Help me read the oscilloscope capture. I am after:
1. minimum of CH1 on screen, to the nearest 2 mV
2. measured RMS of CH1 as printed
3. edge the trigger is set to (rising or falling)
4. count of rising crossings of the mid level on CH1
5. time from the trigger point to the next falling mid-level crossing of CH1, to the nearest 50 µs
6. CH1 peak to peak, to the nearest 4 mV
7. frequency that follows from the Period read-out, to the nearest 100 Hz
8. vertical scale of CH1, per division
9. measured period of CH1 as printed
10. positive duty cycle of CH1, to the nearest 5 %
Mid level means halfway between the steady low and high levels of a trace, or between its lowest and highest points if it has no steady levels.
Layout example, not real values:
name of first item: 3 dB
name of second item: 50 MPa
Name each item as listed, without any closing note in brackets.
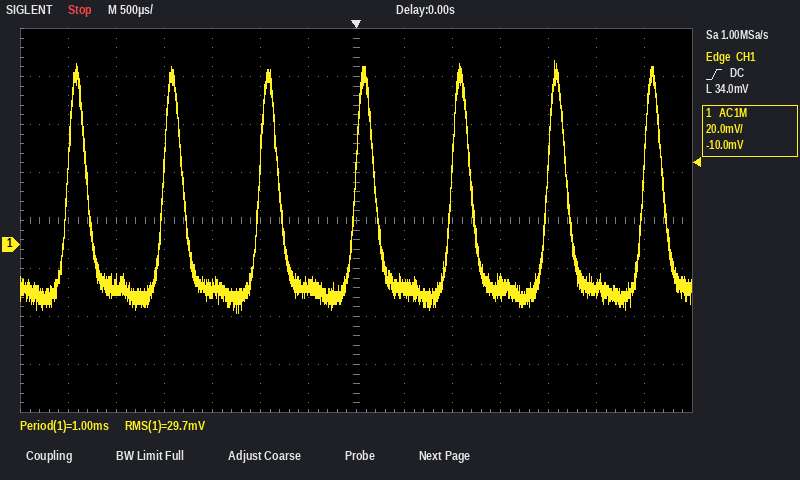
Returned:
minimum of CH1 on screen, to the nearest 2 mV: -28 mV
measured RMS of CH1 as printed: 29.7 mV
edge the trigger is set to: rising
count of rising crossings of the mid level on CH1: 7
time from the trigger point to the next falling mid-level crossing of CH1, to the nearest 50 µs: 200 µs
CH1 peak to peak, to the nearest 4 mV: 104 mV
frequency that follows from the Period read-out, to the nearest 100 Hz: 1.0 kHz
vertical scale of CH1, per division: 20 mV
measured period of CH1 as printed: 1.00 ms
positive duty cycle of CH1, to the nearest 5 %: 20 %
